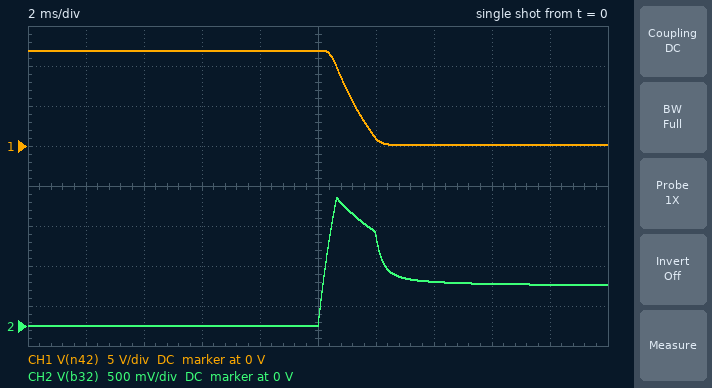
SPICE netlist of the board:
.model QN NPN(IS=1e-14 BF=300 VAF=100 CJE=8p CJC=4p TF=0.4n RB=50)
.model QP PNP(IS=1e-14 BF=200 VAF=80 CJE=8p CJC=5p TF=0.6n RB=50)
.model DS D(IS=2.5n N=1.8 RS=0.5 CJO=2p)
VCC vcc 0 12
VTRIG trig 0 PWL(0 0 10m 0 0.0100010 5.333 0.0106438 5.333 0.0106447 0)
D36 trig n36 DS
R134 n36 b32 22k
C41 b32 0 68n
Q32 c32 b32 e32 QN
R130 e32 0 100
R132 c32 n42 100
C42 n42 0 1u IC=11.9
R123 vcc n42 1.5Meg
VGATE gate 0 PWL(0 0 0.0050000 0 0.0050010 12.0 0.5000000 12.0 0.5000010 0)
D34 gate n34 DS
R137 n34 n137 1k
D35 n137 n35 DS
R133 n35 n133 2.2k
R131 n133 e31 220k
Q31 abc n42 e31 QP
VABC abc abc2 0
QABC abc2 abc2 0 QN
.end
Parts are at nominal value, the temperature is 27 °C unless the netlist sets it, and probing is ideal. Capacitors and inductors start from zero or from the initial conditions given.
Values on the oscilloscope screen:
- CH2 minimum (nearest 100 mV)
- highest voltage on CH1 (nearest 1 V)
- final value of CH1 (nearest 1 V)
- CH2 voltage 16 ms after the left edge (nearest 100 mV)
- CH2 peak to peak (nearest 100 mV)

0 V
12 V
0 V
500 mV
1.6 V
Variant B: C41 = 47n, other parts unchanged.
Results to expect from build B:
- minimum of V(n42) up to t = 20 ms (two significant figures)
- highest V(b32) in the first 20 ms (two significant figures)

72 mV
2.0 V
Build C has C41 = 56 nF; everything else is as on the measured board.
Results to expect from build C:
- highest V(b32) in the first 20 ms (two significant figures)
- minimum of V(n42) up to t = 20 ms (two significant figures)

1.8 V
68 mV
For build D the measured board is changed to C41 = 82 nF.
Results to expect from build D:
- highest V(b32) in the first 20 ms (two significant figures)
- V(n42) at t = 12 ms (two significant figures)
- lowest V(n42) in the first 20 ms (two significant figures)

1.4 V
3.2 V
60 mV
